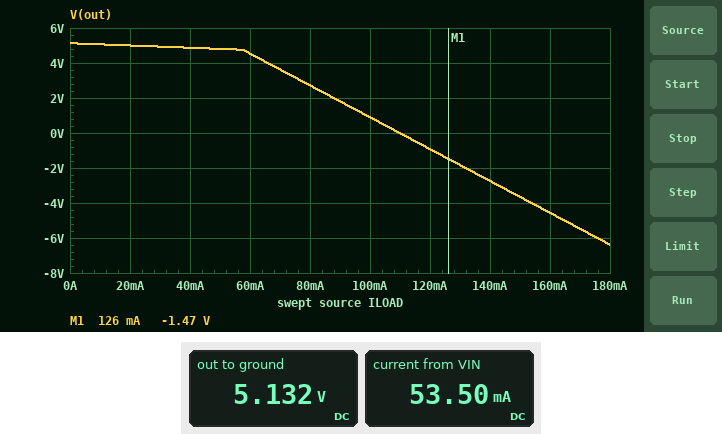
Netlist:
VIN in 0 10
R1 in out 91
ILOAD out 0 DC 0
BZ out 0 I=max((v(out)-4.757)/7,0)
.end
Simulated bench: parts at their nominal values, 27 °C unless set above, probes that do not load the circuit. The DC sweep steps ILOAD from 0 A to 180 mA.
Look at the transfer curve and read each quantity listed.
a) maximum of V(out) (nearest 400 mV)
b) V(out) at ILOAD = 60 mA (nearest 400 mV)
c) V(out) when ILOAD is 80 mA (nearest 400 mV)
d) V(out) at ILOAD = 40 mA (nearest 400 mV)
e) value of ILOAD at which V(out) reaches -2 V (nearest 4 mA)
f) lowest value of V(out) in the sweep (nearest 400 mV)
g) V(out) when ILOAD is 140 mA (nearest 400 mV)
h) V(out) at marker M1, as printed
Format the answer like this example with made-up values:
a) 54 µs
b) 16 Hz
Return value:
a) 5.2 V
b) 4.4 V
c) 2.8 V
d) 4.8 V
e) 132 mA
f) -6.4 V
g) -2.8 V
h) -1.47 V
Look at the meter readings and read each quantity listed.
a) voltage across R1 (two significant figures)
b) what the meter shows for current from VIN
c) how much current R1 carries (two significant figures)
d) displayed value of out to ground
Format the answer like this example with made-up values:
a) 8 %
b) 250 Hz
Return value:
a) 4.9 V
b) 53.50 mA
c) 53 mA
d) 5.132 V
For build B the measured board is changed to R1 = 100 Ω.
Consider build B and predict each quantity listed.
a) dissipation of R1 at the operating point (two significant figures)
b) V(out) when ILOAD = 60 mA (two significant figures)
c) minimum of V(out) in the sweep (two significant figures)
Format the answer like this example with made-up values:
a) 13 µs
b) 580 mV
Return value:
a) 240 mW
b) 4.0 V
c) -8.0 V
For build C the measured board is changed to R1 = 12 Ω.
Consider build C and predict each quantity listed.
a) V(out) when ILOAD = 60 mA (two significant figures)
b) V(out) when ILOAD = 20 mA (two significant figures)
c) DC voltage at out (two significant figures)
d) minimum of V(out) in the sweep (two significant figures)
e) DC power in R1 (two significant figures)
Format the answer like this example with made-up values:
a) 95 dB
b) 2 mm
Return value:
a) 6.4 V
b) 6.6 V
c) 6.7 V
d) 5.9 V
e) 910 mW
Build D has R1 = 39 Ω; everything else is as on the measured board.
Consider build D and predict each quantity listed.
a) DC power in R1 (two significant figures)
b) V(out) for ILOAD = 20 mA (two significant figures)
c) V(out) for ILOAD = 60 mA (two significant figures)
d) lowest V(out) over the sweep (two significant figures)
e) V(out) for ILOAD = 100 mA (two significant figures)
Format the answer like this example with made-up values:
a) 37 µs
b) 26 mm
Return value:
a) 510 mW
b) 5.4 V
c) 5.2 V
d) 3.0 V
e) 5.0 V
